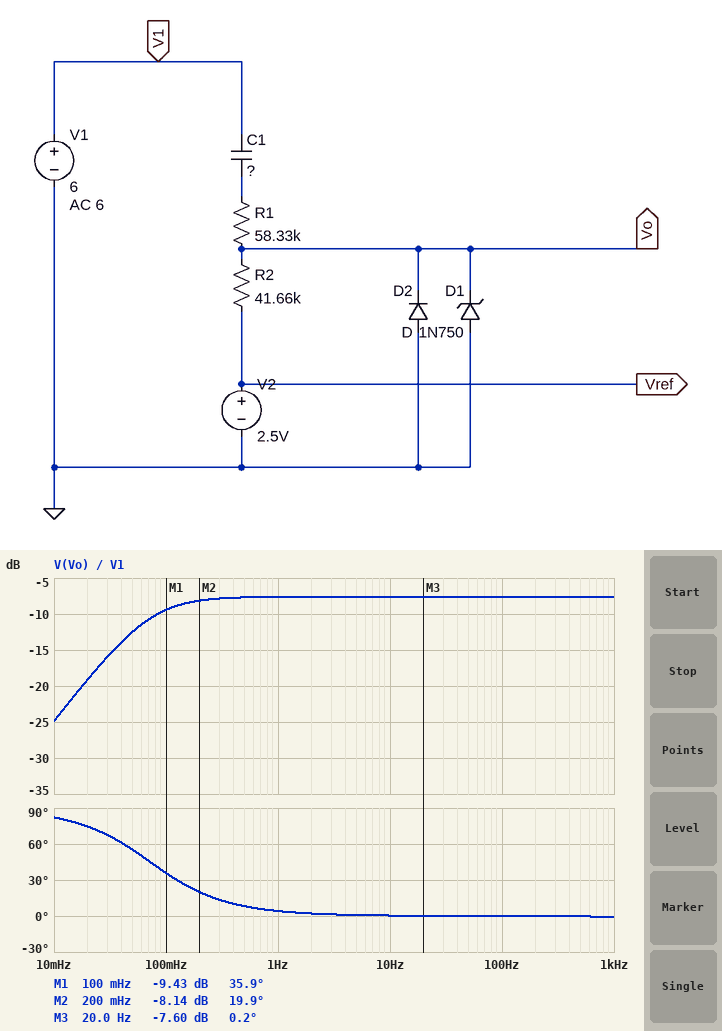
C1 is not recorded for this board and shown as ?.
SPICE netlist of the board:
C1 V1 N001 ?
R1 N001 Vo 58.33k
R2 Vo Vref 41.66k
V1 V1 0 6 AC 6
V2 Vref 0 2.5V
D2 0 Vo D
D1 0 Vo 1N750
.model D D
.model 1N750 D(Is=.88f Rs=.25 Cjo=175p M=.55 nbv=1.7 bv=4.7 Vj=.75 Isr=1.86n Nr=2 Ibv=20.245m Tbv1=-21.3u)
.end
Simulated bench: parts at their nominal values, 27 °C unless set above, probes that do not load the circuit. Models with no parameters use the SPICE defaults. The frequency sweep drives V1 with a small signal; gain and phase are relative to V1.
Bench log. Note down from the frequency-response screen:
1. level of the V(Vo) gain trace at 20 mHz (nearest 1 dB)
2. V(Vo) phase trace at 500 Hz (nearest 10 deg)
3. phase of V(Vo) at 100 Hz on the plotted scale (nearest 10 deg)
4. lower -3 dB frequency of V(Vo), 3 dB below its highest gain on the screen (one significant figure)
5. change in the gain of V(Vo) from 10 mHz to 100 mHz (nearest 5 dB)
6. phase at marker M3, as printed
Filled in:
-19 dB
0 deg
0 deg
70 mHz
15 dB
0.2 deg
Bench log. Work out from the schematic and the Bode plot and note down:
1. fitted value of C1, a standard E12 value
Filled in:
22 µF
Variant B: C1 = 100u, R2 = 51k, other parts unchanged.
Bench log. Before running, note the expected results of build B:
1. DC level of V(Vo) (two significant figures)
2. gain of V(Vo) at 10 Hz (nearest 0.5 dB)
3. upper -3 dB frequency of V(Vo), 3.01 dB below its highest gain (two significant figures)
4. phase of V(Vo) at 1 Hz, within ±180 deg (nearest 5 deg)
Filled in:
2.5 V
-6.5 dB
75 kHz
0 deg
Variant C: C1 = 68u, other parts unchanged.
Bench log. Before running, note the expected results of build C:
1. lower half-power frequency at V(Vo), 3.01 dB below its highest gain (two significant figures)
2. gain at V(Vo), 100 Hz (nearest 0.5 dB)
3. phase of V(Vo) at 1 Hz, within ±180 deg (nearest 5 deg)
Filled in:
23 mHz
-7.5 dB
0 deg
